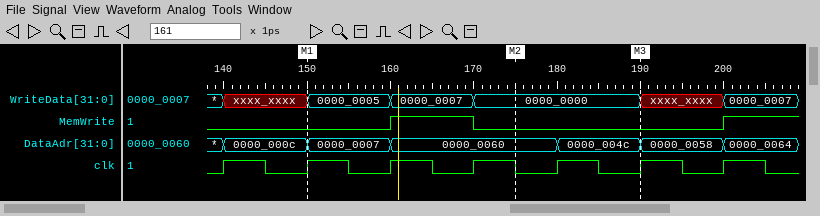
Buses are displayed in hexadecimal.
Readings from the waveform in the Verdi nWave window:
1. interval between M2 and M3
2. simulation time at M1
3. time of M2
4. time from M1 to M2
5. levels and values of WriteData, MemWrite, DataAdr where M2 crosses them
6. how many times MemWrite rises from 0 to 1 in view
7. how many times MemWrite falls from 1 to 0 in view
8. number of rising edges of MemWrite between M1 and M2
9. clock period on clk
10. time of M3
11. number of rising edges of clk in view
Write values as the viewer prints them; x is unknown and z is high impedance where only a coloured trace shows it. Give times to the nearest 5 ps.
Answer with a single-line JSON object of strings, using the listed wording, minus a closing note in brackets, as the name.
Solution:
{"interval between M2 and M3": "15 ps", "simulation time at M1": "150 ps", "time of M2": "175 ps", "time from M1 to M2": "25 ps", "levels and values of WriteData, MemWrite, DataAdr where M2 crosses them": "WriteData=0000_0000, MemWrite=0, DataAdr=0000_0060", "how many times MemWrite rises from 0 to 1 in view": "2", "how many times MemWrite falls from 1 to 0 in view": "1", "number of rising edges of MemWrite between M1 and M2": "1", "clock period on clk": "10 ps", "time of M3": "190 ps", "number of rising edges of clk in view": "7"}
